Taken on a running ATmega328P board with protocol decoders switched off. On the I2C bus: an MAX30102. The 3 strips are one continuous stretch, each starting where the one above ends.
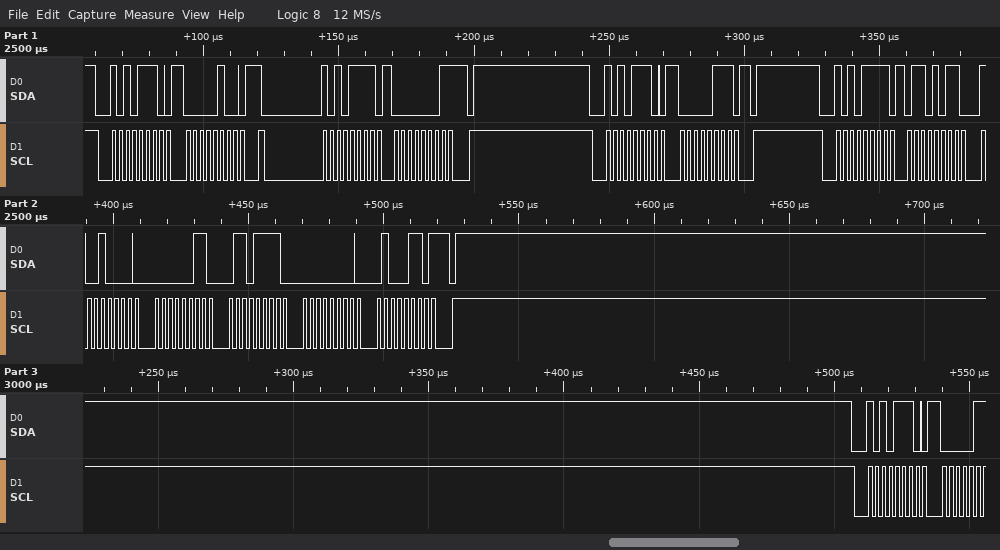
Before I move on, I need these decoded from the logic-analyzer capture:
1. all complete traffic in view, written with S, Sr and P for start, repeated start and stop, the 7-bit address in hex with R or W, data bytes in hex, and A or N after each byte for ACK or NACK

S 57W A 04 A Sr 57R A 01 N P S 57W A 07 A P S 57R A 6B A 90 A 03 A 6F A 00 A 46 N P S 57W A
